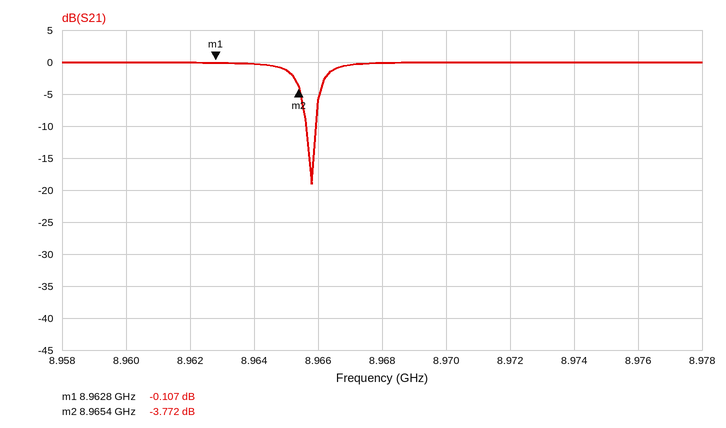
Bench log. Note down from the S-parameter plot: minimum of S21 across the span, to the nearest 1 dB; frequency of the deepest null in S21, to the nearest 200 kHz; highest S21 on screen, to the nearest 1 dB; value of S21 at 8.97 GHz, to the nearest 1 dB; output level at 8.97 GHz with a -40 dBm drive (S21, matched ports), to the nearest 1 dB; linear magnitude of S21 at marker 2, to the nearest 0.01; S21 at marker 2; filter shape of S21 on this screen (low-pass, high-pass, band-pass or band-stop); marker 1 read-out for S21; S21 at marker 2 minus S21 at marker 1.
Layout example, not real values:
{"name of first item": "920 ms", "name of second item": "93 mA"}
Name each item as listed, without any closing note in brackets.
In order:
{"minimum of S21 across the span, to the nearest 1 dB": "-19 dB", "frequency of the deepest null in S21, to the nearest 200 kHz": "8.9658 GHz", "highest S21 on screen, to the nearest 1 dB": "0 dB", "value of S21 at 8.97 GHz, to the nearest 1 dB": "0 dB", "output level at 8.97 GHz with a -40 dBm drive (S21, matched ports), to the nearest 1 dB": "-40 dBm", "linear magnitude of S21 at marker 2, to the nearest 0.01": "0.65", "S21 at marker 2": "-3.772 dB", "filter shape of S21 on this screen": "band-stop", "marker 1 read-out for S21": "-0.107 dB", "S21 at marker 2 minus S21 at marker 1": "-3.665 dB"}
